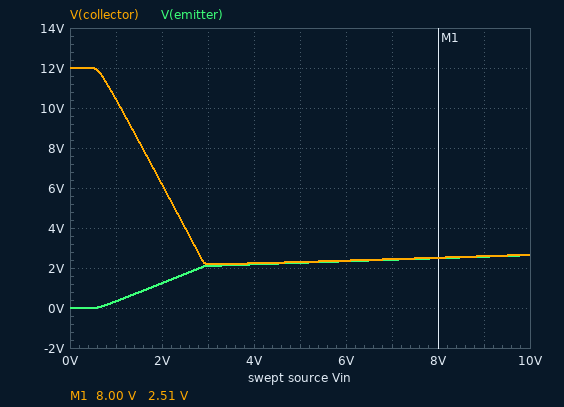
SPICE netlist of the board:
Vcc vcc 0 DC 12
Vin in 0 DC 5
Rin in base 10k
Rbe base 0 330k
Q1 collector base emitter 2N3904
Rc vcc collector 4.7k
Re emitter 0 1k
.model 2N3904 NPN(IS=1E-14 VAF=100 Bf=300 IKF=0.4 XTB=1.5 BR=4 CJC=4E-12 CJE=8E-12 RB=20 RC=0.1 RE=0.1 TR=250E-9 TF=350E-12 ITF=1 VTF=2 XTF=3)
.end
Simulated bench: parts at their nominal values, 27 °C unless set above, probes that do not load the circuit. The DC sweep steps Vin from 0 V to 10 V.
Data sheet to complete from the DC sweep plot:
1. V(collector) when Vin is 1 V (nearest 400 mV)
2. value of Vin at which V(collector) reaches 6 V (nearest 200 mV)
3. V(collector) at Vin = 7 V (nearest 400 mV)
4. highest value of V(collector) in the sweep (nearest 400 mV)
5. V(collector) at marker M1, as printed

10.4 V
2.0 V
2.4 V
12.0 V
2.51 V
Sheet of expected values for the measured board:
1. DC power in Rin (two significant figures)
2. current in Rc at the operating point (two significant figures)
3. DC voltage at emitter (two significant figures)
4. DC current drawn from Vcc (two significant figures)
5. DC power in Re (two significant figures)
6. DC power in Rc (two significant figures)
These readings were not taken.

420 µW
2.1 mA
2.3 V
2.1 mA
5.1 mW
20 mW
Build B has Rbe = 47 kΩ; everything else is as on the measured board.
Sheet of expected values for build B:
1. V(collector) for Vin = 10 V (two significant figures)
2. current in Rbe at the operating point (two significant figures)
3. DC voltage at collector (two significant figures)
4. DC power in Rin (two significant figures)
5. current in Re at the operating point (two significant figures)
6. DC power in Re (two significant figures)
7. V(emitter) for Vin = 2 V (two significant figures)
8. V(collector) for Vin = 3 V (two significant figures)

2.6 V
62 µA
2.3 V
440 µW
2.2 mA
4.9 mW
970 mV
3.8 V
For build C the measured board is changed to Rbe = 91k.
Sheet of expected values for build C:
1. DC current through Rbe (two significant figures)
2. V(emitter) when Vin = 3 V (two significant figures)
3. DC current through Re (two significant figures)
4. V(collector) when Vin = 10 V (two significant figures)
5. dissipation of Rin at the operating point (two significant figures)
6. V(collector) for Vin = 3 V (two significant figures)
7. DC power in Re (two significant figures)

32 µA
2.0 V
2.2 mA
2.6 V
430 µW
2.8 V
5.0 mW
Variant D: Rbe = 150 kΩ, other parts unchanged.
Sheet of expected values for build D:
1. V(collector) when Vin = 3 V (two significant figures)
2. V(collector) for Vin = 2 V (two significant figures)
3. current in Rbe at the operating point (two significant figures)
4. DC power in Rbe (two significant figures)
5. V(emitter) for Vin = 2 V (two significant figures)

2.3 V
6.5 V
20 µA
58 µW
1.2 V
